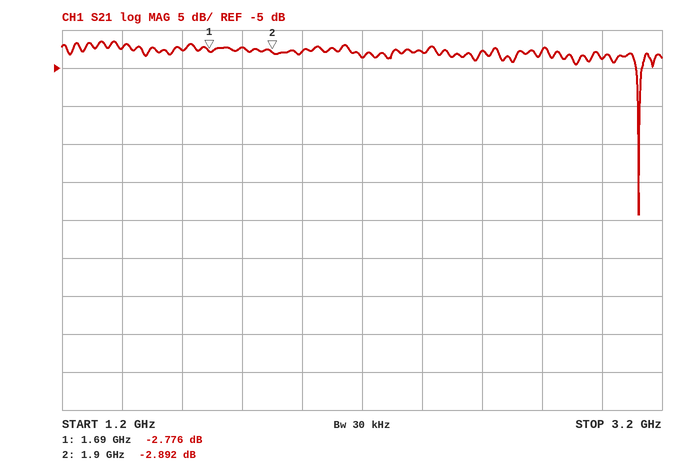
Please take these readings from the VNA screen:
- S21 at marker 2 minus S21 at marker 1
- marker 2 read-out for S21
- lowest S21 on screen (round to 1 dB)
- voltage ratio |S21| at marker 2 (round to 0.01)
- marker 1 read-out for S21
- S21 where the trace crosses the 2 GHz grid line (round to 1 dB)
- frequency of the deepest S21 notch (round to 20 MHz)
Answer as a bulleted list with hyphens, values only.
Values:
- -0.116 dB
- -2.892 dB
- -24 dB
- 0.72
- -2.776 dB
- -3 dB
- 3.12 GHz
